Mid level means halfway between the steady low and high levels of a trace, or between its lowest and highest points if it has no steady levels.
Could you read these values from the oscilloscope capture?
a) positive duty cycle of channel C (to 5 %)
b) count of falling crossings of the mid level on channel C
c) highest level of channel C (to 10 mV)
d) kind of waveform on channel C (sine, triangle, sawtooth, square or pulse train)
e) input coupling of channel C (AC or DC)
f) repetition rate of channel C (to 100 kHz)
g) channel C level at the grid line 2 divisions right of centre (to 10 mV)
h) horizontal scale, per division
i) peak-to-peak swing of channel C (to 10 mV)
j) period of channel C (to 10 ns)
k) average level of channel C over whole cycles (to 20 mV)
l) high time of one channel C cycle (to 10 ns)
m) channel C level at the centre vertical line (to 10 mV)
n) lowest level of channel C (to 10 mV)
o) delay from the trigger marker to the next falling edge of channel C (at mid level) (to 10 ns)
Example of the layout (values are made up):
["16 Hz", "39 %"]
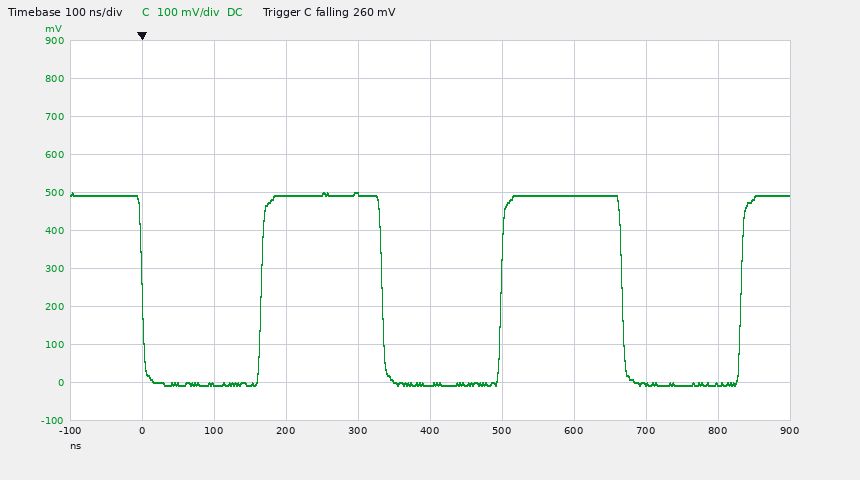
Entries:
["50 %", "3", "500 mV", "square", "DC", "3.0 MHz", "490 mV", "100 ns", "510 mV", "330 ns", "240 mV", "170 ns", "-10 mV", "-10 mV", "330 ns"]
